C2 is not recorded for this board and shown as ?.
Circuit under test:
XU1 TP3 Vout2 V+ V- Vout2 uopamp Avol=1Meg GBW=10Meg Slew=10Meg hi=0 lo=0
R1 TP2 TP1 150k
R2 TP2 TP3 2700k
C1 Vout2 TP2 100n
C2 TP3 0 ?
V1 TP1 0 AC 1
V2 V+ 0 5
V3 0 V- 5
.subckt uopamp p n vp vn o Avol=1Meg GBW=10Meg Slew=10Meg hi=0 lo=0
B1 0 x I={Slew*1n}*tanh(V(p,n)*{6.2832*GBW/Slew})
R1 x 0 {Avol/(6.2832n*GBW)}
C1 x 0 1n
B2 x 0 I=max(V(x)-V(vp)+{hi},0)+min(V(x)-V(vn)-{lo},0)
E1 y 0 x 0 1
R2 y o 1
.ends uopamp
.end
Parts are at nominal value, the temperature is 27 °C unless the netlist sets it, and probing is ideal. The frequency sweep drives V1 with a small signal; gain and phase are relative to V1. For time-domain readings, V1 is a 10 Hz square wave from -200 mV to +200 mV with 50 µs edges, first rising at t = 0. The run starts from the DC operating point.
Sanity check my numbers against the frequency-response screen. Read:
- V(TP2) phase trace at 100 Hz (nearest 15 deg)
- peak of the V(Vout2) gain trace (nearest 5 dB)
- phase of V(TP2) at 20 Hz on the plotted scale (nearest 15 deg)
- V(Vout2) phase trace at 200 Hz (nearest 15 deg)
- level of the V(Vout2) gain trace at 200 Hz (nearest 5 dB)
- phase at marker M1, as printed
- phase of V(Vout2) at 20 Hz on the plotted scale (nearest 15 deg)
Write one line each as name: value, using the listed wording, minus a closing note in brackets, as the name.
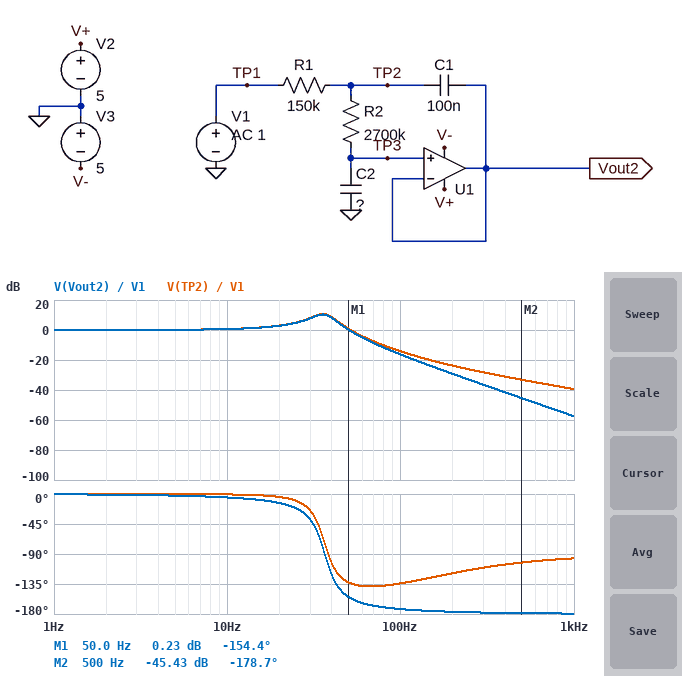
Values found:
V(TP2) phase trace at 100 Hz: -135 deg
peak of the V(Vout2) gain trace: 10 dB
phase of V(TP2) at 20 Hz on the plotted scale: 0 deg
V(Vout2) phase trace at 200 Hz: -180 deg
level of the V(Vout2) gain trace at 200 Hz: -30 dB
phase at marker M1, as printed: -154.4 deg
phase of V(Vout2) at 20 Hz on the plotted scale: -15 deg
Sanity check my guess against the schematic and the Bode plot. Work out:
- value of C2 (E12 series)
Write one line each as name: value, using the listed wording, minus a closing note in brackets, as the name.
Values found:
value of C2: 470 pF
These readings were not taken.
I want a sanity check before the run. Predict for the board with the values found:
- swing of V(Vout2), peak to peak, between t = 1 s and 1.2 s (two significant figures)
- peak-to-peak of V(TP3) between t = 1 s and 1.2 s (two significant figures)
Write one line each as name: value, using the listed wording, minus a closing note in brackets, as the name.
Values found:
swing of V(Vout2), peak to peak, between t = 1 s and 1.2 s: 870 mV
peak-to-peak of V(TP3) between t = 1 s and 1.2 s: 870 mV
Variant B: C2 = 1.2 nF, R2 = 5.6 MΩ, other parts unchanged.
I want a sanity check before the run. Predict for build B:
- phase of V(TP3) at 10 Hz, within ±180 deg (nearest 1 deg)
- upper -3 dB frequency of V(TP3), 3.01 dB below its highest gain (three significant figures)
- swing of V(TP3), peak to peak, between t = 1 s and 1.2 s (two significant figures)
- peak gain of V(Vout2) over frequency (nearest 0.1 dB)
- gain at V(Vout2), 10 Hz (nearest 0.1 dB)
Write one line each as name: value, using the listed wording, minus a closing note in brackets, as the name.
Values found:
phase of V(TP3) at 10 Hz, within ±180 deg: -36 deg
upper -3 dB frequency of V(TP3), 3.01 dB below its highest gain: 18.8 Hz
swing of V(TP3), peak to peak, between t = 1 s and 1.2 s: 670 mV
peak gain of V(Vout2) over frequency: 3.8 dB
gain at V(Vout2), 10 Hz: 2.6 dB
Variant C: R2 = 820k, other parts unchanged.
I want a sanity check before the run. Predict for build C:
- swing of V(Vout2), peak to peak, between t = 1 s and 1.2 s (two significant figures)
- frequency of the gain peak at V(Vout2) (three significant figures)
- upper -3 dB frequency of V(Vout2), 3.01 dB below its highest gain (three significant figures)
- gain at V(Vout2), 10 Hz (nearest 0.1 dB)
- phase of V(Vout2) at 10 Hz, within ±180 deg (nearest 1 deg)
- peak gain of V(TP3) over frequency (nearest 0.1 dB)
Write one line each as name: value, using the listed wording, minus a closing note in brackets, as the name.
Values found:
swing of V(Vout2), peak to peak, between t = 1 s and 1.2 s: 1.0 V
frequency of the gain peak at V(Vout2): 65.6 Hz
upper -3 dB frequency of V(Vout2), 3.01 dB below its highest gain: 71.6 Hz
gain at V(Vout2), 10 Hz: 0.2 dB
phase of V(Vout2) at 10 Hz, within ±180 deg: -2 deg
peak gain of V(TP3) over frequency: 14.5 dB
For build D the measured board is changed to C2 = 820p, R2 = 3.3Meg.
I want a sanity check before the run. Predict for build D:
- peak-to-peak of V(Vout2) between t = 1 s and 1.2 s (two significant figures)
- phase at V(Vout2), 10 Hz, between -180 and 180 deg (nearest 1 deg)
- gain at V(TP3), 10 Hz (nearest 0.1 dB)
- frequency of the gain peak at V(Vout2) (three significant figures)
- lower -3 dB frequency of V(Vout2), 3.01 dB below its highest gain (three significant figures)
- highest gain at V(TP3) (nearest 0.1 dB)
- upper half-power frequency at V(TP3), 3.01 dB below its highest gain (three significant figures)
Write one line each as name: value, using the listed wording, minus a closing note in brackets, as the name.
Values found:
peak-to-peak of V(Vout2) between t = 1 s and 1.2 s: 760 mV
phase at V(Vout2), 10 Hz, between -180 and 180 deg: -12 deg
gain at V(TP3), 10 Hz: 1.3 dB
frequency of the gain peak at V(Vout2): 23.7 Hz
lower -3 dB frequency of V(Vout2), 3.01 dB below its highest gain: 17.1 Hz
highest gain at V(TP3): 7.3 dB
upper half-power frequency at V(TP3), 3.01 dB below its highest gain: 28.9 Hz
